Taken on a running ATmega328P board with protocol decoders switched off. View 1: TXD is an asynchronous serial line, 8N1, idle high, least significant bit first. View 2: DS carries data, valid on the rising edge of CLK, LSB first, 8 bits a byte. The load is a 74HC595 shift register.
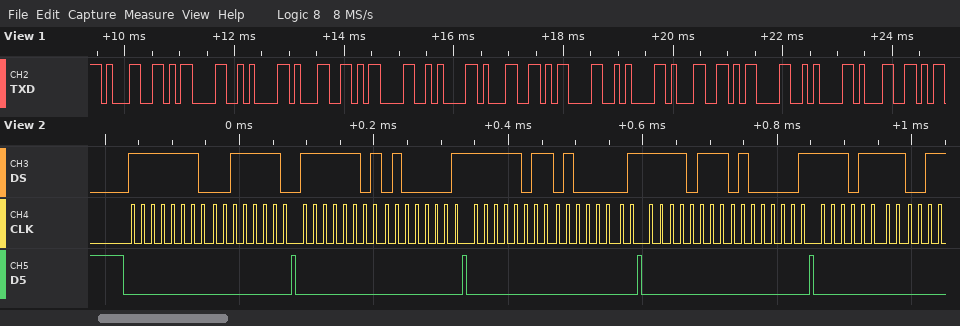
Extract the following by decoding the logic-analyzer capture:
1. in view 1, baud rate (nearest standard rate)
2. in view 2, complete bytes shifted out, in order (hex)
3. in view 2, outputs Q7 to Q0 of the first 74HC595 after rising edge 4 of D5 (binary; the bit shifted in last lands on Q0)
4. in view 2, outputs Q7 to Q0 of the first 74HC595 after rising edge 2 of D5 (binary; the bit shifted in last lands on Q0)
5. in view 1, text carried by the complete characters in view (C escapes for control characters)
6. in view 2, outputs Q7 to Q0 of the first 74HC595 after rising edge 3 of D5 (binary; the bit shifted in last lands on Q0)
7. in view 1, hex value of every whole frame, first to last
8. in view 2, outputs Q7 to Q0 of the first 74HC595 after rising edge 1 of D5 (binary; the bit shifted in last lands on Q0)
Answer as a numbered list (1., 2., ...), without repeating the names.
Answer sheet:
1. 9600 baud
2. 7F 7C BF 82 DF 82 EF 82 F7
3. 01000001
4. 01000001
5. "1\r\n1\r\n1\r\n1\r\n1"
6. 01000001
7. 31 0D 0A 31 0D 0A 31 0D 0A 31 0D 0A 31
8. 00111110
